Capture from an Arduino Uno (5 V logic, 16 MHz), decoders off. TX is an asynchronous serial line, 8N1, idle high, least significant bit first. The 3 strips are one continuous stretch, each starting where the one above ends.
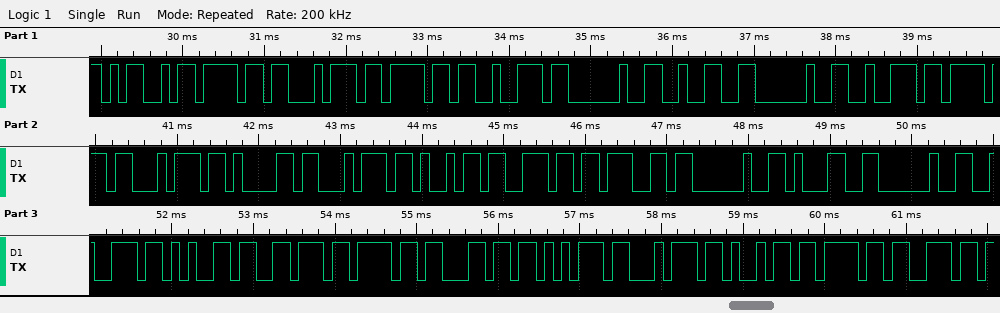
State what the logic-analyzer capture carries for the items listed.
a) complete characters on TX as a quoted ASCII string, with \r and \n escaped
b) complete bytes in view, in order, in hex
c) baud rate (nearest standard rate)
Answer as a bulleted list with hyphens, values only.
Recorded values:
- "Motor 2 rotating 1 revolution"
- 0x4D 0x6F 0x74 0x6F 0x72 0x20 0x32 0x20 0x72 0x6F 0x74 0x61 0x74 0x69 0x6E 0x67 0x20 0x31 0x20 0x72 0x65 0x76 0x6F 0x6C 0x75 0x74 0x69 0x6F 0x6E
- 9600 baud
